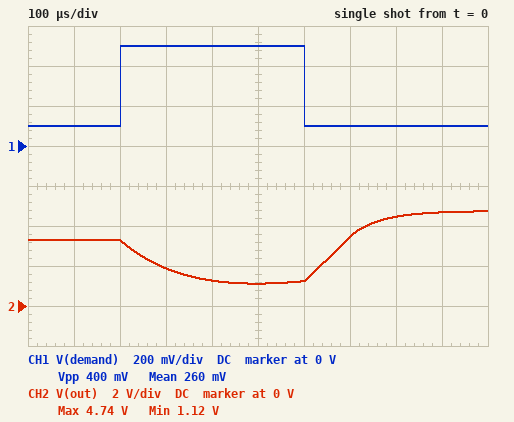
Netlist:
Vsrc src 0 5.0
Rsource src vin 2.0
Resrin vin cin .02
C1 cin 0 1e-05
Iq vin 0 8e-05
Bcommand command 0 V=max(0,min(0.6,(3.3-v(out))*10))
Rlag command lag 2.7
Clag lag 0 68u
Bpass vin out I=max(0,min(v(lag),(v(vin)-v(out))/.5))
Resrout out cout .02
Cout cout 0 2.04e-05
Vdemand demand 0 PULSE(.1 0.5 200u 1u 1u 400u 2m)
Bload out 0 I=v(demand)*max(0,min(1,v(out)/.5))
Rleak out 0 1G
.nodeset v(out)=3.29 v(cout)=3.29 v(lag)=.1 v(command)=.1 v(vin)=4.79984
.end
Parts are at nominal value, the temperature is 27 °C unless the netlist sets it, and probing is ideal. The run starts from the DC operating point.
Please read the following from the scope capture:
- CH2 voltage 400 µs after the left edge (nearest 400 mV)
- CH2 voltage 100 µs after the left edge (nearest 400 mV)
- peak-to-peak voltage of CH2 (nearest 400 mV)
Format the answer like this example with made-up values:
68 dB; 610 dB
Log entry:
1.2 V; 3.2 V; 3.6 V
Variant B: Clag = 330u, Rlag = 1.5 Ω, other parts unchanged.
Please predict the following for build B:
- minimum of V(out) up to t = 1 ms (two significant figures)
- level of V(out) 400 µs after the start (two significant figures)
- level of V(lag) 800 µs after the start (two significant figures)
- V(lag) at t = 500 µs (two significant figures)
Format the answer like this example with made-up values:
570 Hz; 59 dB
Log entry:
290 mV; 340 mV; 440 mV; 330 mV
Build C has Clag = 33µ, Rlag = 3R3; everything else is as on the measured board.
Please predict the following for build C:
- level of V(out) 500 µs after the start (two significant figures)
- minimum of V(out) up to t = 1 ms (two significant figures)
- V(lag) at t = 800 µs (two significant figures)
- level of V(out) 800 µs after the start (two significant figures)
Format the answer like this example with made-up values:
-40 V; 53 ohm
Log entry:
2.2 V; 2.0 V; 120 mV; 4.6 V
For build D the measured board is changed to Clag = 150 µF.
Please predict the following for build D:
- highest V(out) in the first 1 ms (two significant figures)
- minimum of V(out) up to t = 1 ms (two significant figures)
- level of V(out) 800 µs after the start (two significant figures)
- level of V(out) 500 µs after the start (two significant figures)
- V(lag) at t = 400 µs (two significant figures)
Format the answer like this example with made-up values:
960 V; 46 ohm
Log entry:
4.7 V; 330 mV; 3.8 V; 350 mV; 290 mV
